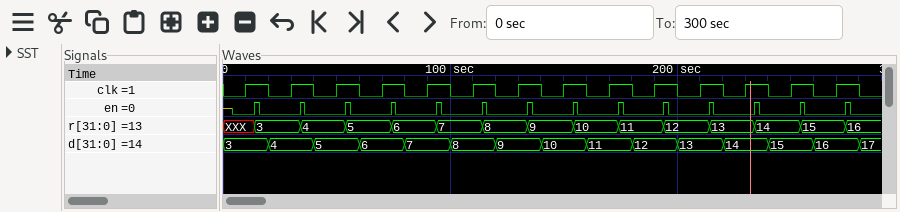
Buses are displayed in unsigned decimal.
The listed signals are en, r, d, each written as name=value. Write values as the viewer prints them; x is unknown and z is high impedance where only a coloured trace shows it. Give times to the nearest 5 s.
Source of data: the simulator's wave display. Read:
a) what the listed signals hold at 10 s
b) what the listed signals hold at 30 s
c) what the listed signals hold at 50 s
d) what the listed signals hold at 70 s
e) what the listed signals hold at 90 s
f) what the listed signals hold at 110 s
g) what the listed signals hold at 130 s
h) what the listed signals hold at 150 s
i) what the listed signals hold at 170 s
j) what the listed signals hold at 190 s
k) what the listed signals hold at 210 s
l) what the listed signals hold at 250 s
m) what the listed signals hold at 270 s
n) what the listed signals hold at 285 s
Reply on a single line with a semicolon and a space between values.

en=0, r=XXX, d=3; en=0, r=3, d=4; en=0, r=4, d=5; en=0, r=5, d=6; en=0, r=6, d=7; en=0, r=7, d=8; en=0, r=8, d=9; en=0, r=9, d=10; en=0, r=10, d=11; en=0, r=11, d=12; en=0, r=12, d=13; en=0, r=14, d=15; en=0, r=15, d=16; en=0, r=16, d=17
